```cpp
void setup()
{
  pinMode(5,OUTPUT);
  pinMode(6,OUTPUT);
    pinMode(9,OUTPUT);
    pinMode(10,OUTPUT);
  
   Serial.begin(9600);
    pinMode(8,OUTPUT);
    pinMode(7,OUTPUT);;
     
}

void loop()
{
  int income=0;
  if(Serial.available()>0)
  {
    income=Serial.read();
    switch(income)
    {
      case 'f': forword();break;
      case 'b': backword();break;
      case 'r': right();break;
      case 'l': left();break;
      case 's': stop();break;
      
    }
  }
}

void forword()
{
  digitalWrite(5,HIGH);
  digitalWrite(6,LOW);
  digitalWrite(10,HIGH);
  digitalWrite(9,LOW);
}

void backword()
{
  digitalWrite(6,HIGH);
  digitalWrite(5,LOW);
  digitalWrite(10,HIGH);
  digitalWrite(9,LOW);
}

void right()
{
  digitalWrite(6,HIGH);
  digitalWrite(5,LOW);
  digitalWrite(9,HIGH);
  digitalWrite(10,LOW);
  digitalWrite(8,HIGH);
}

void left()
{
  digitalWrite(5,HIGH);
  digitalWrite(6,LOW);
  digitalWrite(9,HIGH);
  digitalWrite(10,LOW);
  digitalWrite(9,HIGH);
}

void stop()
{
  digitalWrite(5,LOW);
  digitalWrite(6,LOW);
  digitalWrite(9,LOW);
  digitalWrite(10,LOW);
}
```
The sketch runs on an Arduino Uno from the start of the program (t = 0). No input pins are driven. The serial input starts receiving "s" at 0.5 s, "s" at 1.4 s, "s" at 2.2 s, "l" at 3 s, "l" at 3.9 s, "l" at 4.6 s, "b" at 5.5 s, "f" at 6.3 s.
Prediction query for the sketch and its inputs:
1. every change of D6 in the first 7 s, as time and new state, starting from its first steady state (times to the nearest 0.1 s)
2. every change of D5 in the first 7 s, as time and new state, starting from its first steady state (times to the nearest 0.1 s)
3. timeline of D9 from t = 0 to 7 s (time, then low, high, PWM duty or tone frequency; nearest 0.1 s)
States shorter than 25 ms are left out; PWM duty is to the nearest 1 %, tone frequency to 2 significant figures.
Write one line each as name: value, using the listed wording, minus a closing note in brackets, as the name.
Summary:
every change of D6 in the first 7 s, as time and new state, starting from its first steady state: 0 s low; 5.5 s high; 6.3 s low
every change of D5 in the first 7 s, as time and new state, starting from its first steady state: 0 s low; 3 s high; 5.5 s low; 6.3 s high
timeline of D9 from t = 0 to 7 s: 0 s low; 3 s high; 5.5 s low
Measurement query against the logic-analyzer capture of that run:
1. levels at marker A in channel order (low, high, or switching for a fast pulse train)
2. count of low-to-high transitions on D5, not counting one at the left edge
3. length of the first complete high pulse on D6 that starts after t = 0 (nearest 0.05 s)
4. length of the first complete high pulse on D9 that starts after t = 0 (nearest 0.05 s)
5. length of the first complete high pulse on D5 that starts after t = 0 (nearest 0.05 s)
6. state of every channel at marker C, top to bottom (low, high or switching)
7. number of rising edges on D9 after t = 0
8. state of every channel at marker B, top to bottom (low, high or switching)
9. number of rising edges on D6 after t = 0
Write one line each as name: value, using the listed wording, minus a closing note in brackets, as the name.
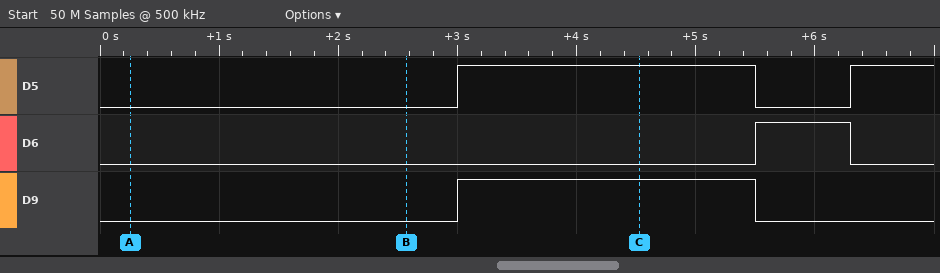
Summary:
levels at marker A in channel order: D5 low, D6 low, D9 low
count of low-to-high transitions on D5, not counting one at the left edge: 2
length of the first complete high pulse on D6 that starts after t = 0: 0.80 s
length of the first complete high pulse on D9 that starts after t = 0: 2.50 s
length of the first complete high pulse on D5 that starts after t = 0: 2.50 s
state of every channel at marker C, top to bottom: D5 high, D6 low, D9 high
number of rising edges on D9 after t = 0: 1
state of every channel at marker B, top to bottom: D5 low, D6 low, D9 low
number of rising edges on D6 after t = 0: 1
